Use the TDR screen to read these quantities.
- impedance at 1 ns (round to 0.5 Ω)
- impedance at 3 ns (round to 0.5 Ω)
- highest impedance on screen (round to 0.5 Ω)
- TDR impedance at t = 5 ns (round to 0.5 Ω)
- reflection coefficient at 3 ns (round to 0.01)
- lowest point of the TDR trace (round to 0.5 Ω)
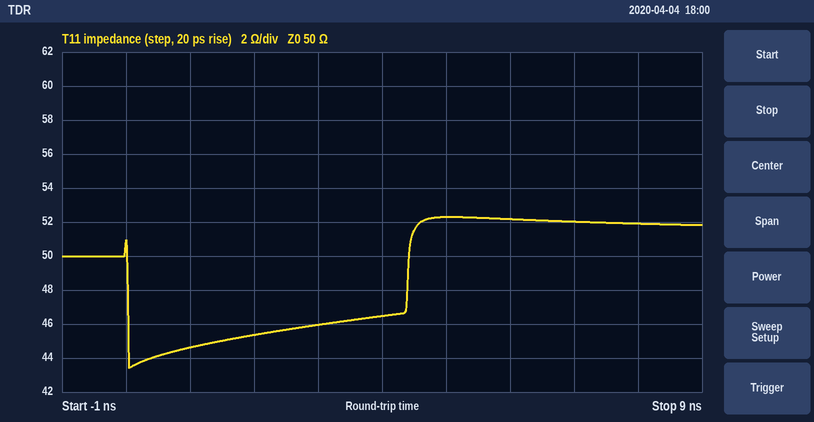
44.5 Ω
46.0 Ω
52.5 Ω
52.5 Ω
-0.04
43.5 Ω
